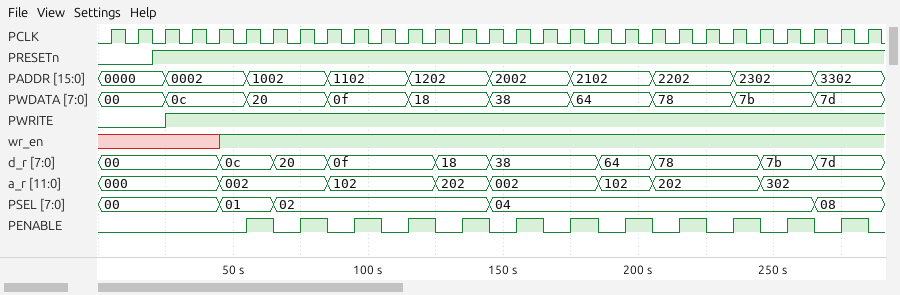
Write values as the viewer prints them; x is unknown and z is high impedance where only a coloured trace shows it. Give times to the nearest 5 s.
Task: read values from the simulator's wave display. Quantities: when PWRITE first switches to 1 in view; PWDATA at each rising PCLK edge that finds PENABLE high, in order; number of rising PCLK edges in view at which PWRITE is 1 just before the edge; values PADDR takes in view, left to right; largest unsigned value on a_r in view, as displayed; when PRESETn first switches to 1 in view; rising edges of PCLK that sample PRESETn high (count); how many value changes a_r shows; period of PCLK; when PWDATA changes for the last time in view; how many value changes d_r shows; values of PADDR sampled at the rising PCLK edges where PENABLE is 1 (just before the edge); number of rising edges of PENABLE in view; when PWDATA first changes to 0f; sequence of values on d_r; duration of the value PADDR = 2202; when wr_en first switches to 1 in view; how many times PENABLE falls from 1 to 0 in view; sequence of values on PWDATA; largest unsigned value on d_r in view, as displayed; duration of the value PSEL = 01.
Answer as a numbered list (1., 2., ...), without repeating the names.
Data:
1. 25 s
2. 20, 20, 0f, 18, 18, 38, 64, 64, 78, 7b, 7b, 7d
3. 26
4. 0000, 0002, 1002, 1102, 1202, 2002, 2102, 2202, 2302, 3302
5. 302
6. 20 s
7. 27
8. 7
9. 10 s
10. 265 s
11. 9
12. 1002, 1002, 1102, 1202, 1202, 2002, 2102, 2102, 2202, 2302, 2302, 3302
13. 12
14. 85 s
15. 00, 0c, 20, 0f, 18, 38, 64, 78, 7b, 7d
16. 30 s
17. 45 s
18. 12
19. 00, 0c, 20, 0f, 18, 38, 64, 78, 7b, 7d
20. 7d
21. 20 s
